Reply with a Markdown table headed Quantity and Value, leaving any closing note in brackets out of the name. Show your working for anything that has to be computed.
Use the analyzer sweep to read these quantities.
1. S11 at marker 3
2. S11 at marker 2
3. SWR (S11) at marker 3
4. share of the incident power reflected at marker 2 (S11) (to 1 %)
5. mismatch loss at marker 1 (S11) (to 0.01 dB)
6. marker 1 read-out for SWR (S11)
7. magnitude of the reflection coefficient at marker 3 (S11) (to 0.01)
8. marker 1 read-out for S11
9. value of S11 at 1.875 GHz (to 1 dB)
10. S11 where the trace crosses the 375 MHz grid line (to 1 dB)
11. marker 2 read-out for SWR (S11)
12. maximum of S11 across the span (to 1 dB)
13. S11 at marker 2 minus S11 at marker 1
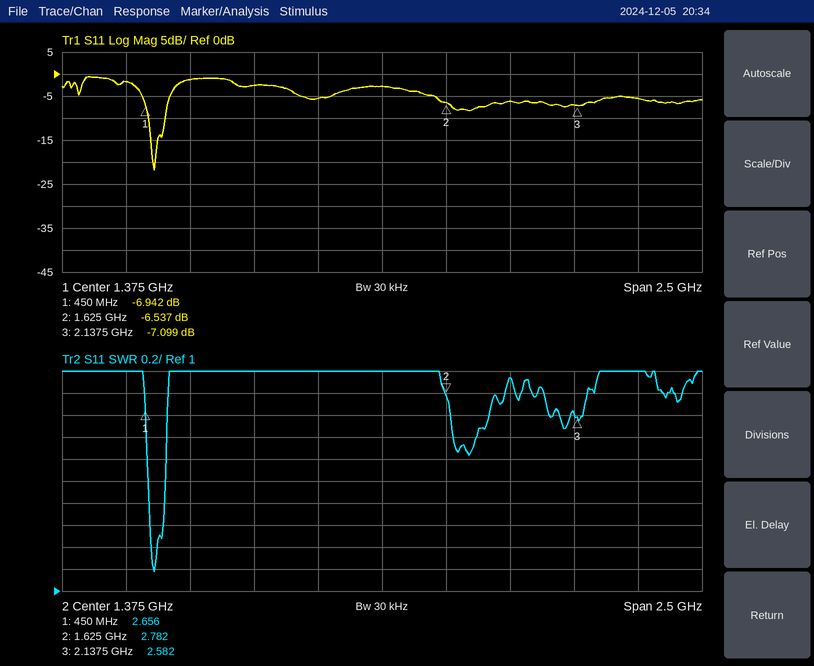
| Quantity | Value |
|---|---|
| S11 at marker 3 | -7.099 dB |
| S11 at marker 2 | -6.537 dB |
| SWR (S11) at marker 3 | 2.582 |
| share of the incident power reflected at marker 2 (S11) | 10^(-6.537/10) ≈ 22 % |
| mismatch loss at marker 1 (S11) | −10 log10(1 − 10^(-6.942/10)) ≈ 0.98 dB |
| marker 1 read-out for SWR | 2.656 |
| magnitude of the reflection coefficient at marker 3 (S11) | 10^(-7.099/20) ≈ 0.44 |
| marker 1 read-out for S11 | -6.942 dB |
| value of S11 at 1.875 GHz | -6 dB |
| S11 where the trace crosses the 375 MHz grid line | -2 dB |
| marker 2 read-out for SWR | 2.782 |
| maximum of S11 across the span | -1 dB |
| S11 at marker 2 minus S11 at marker 1 | -6.537 − (-6.942) = 0.405 dB |
